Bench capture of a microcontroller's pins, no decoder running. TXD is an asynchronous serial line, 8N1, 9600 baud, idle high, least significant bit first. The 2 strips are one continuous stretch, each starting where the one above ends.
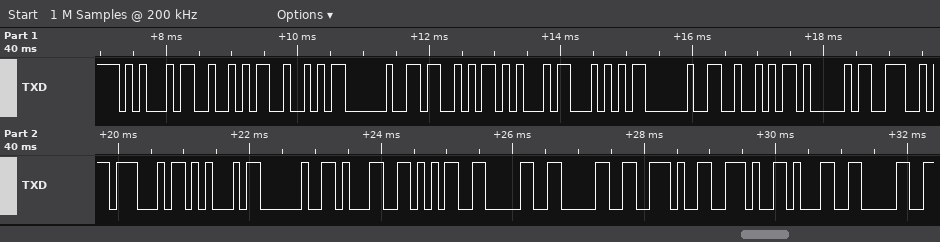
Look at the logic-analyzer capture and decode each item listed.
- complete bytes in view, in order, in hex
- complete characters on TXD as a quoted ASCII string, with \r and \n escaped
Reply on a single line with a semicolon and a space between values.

0x45 0x52 0x52 0x20 0x53 0x45 0x54 0x20 0x52 0x41 0x4E 0x47 0x45 0x20 0x31 0x35 0x30 0x30 0x2E 0x2E 0x31 0x30; "ERR SET RANGE 1500..10"
